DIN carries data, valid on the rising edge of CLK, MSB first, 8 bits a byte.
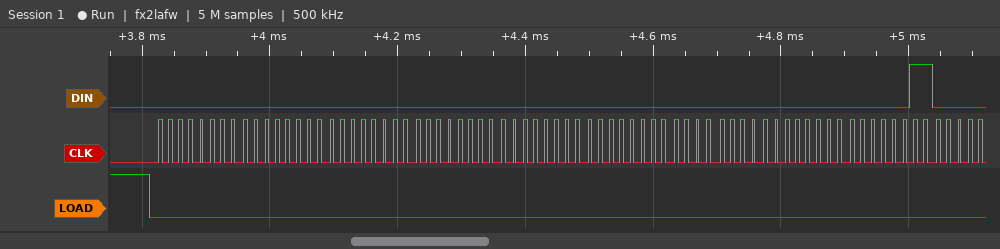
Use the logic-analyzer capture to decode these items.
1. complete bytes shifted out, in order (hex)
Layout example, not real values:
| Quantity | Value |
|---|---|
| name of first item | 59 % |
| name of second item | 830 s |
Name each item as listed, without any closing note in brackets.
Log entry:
| Quantity | Value |
|---|---|
| complete bytes shifted out, in order | 0x00 0x00 0x00 0x00 0x00 0x00 0x00 0x00 0x03 |
